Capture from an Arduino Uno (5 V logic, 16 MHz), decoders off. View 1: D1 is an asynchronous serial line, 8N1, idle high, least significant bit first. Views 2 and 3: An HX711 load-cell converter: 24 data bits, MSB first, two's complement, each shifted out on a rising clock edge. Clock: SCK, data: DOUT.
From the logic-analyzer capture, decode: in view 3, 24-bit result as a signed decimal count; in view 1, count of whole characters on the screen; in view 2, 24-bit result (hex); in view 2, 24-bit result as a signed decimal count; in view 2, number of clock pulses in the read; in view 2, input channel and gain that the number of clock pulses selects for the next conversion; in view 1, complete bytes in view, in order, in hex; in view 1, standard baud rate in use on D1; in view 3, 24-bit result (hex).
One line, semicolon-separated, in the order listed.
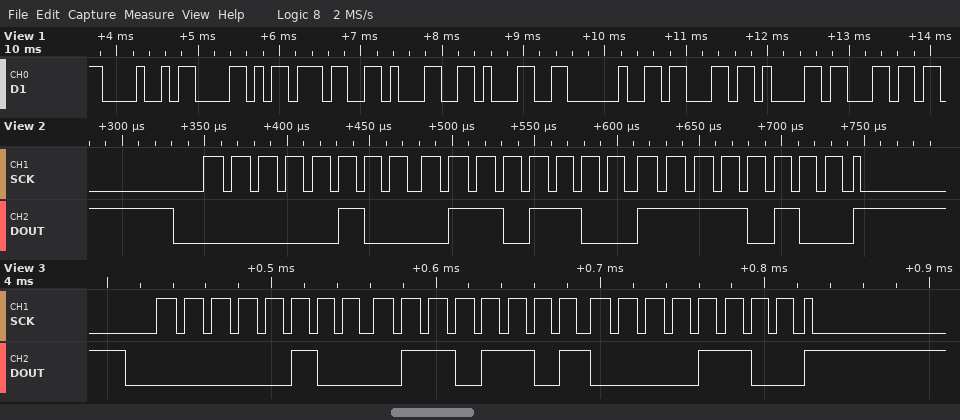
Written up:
290060; 9; 0x046CF4; 290036; 25; channel A, gain 128; 48 58 37 31 31 20 63 61 6C; 9600 baud; 0x046D0C
